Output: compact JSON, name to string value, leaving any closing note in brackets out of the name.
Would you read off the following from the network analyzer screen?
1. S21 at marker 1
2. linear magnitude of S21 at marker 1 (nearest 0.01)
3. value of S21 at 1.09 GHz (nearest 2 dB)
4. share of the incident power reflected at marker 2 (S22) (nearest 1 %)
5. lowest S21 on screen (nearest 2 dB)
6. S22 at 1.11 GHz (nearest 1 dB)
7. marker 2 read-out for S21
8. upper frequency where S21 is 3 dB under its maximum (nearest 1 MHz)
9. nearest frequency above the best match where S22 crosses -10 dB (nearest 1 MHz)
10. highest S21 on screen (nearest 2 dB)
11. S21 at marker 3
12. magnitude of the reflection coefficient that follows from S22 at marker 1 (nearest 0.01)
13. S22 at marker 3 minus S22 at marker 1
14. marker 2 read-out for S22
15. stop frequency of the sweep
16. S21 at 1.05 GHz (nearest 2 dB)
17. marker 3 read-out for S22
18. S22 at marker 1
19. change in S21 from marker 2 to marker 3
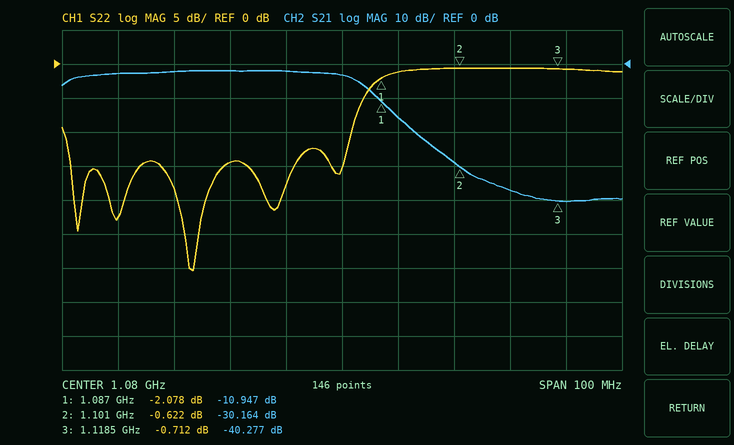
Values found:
{"S21 at marker 1": "-10.947 dB", "linear magnitude of S21 at marker 1": "0.28", "value of S21 at 1.09 GHz": "-16 dB", "share of the incident power reflected at marker 2 (S22)": "87 %", "lowest S21 on screen": "-40 dB", "S22 at 1.11 GHz": "-1 dB", "marker 2 read-out for S21": "-30.164 dB", "upper frequency where S21 is 3 dB under its maximum": "1.083 GHz", "nearest frequency above the best match where S22 crosses -10 dB": "1.082 GHz", "highest S21 on screen": "-2 dB", "S21 at marker 3": "-40.277 dB", "magnitude of the reflection coefficient that follows from S22 at marker 1": "0.79", "S22 at marker 3 minus S22 at marker 1": "1.366 dB", "marker 2 read-out for S22": "-0.622 dB", "stop frequency of the sweep": "1.13 GHz", "S21 at 1.05 GHz": "-2 dB", "marker 3 read-out for S22": "-0.712 dB", "S22 at marker 1": "-2.078 dB", "change in S21 from marker 2 to marker 3": "-10.113 dB"}
